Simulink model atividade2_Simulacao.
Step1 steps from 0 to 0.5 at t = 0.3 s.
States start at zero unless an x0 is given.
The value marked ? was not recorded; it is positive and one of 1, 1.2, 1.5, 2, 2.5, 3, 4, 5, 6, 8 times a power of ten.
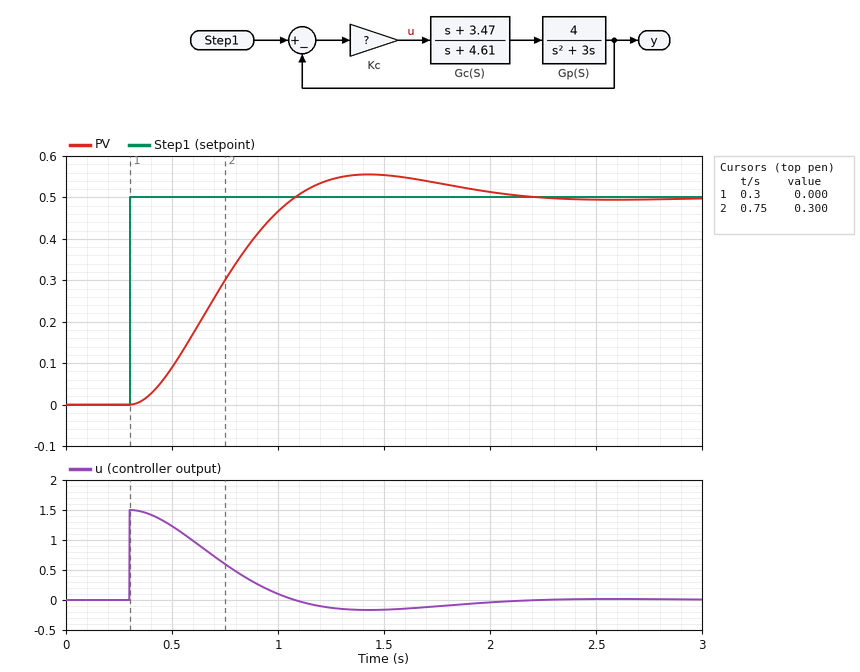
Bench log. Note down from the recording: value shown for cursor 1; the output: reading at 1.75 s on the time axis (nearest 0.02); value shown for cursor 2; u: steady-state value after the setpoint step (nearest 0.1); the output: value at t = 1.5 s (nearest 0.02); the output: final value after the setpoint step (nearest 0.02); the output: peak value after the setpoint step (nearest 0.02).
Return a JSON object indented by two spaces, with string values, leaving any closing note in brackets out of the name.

{
  "value shown for cursor 1": "0.000",
  "the output: reading at 1.75 s on the time axis": "0.54",
  "value shown for cursor 2": "0.300",
  "u: steady-state value after the setpoint step": "0.0",
  "the output: value at t = 1.5 s": "0.56",
  "the output: final value after the setpoint step": "0.50",
  "the output: peak value after the setpoint step": "0.56"
}
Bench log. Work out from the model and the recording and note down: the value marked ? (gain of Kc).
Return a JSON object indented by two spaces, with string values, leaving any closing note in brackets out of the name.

{
  "the value marked ?": "3"
}
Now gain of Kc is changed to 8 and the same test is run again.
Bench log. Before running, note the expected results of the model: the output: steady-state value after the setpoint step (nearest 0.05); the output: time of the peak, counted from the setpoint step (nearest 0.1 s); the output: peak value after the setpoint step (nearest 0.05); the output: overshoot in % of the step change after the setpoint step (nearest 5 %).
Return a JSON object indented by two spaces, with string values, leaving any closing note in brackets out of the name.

{
  "the output: steady-state value after the setpoint step": "0.50",
  "the output: time of the peak, counted from the setpoint step": "0.6 s",
  "the output: peak value after the setpoint step": "0.65",
  "the output: overshoot in % of the step change after the setpoint step": "30 %"
}
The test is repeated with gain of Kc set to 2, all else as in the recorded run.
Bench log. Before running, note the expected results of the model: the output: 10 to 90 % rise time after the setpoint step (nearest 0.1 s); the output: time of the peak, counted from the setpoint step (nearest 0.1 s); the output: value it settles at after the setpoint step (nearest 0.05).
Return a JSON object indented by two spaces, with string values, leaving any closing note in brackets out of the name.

{
  "the output: 10 to 90 % rise time after the setpoint step": "0.8 s",
  "the output: time of the peak, counted from the setpoint step": "1.6 s",
  "the output: value it settles at after the setpoint step": "0.50"
}
